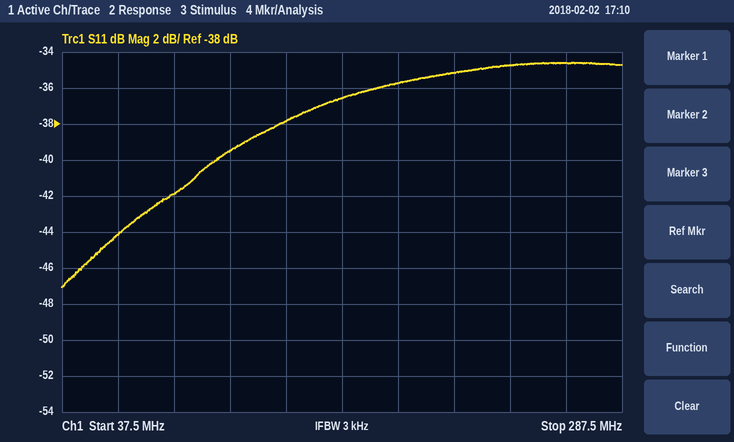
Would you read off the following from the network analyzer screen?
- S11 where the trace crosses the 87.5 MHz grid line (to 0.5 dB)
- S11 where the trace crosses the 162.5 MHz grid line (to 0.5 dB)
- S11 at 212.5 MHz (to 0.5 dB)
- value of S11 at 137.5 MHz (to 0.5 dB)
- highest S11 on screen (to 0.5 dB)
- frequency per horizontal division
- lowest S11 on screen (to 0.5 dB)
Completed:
-42.0 dB
-36.5 dB
-35.0 dB
-38.0 dB
-34.5 dB
25 MHz
-47.0 dB
